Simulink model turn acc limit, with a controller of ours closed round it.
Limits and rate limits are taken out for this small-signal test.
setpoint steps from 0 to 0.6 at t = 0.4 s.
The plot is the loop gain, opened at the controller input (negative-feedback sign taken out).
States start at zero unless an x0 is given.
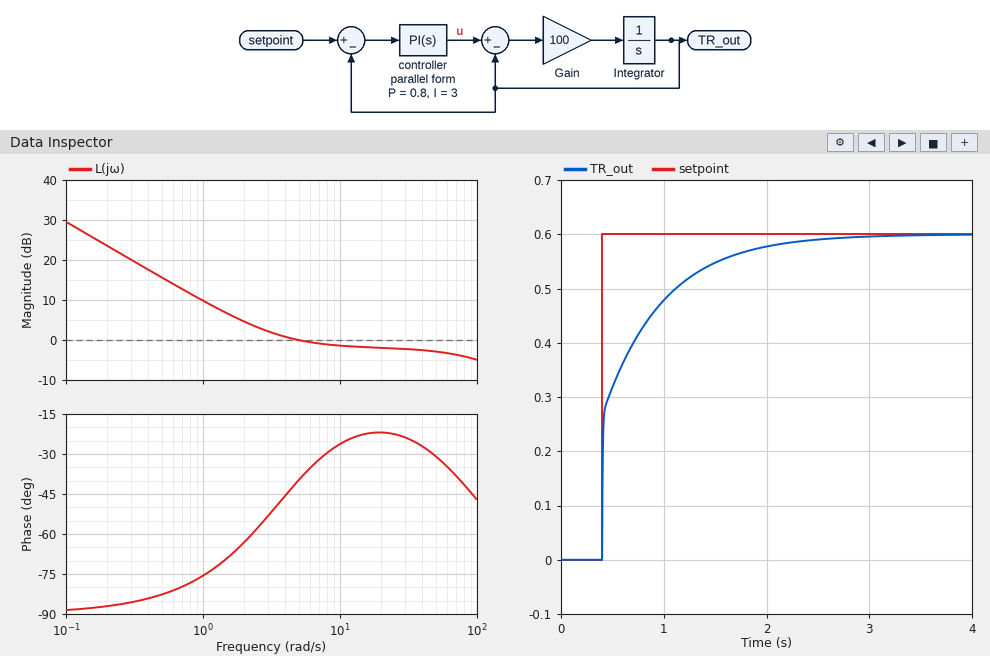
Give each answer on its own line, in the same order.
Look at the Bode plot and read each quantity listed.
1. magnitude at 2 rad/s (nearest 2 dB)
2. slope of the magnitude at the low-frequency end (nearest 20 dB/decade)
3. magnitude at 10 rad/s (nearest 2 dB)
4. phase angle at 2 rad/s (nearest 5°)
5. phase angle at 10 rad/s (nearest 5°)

4 dB
-20 dB/decade
-2 dB
-65°
-25°
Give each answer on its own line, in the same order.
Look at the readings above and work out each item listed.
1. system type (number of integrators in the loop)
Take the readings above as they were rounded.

1
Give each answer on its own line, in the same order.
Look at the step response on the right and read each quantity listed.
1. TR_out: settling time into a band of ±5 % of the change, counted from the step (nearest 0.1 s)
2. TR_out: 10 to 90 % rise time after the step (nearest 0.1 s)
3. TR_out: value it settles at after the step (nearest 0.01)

1.4 s
1.0 s
0.60
